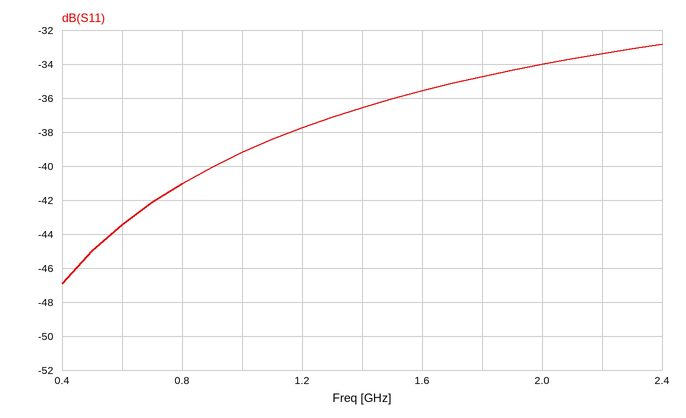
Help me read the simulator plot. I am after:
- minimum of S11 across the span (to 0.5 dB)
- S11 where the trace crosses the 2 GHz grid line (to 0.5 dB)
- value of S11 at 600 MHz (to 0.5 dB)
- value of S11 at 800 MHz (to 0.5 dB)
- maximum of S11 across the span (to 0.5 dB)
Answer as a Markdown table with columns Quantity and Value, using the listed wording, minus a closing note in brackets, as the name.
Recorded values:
| Quantity | Value |
|---|---|
| minimum of S11 across the span | -47.0 dB |
| S11 where the trace crosses the 2 GHz grid line | -34.0 dB |
| value of S11 at 600 MHz | -43.5 dB |
| value of S11 at 800 MHz | -41.0 dB |
| maximum of S11 across the span | -33.0 dB |
